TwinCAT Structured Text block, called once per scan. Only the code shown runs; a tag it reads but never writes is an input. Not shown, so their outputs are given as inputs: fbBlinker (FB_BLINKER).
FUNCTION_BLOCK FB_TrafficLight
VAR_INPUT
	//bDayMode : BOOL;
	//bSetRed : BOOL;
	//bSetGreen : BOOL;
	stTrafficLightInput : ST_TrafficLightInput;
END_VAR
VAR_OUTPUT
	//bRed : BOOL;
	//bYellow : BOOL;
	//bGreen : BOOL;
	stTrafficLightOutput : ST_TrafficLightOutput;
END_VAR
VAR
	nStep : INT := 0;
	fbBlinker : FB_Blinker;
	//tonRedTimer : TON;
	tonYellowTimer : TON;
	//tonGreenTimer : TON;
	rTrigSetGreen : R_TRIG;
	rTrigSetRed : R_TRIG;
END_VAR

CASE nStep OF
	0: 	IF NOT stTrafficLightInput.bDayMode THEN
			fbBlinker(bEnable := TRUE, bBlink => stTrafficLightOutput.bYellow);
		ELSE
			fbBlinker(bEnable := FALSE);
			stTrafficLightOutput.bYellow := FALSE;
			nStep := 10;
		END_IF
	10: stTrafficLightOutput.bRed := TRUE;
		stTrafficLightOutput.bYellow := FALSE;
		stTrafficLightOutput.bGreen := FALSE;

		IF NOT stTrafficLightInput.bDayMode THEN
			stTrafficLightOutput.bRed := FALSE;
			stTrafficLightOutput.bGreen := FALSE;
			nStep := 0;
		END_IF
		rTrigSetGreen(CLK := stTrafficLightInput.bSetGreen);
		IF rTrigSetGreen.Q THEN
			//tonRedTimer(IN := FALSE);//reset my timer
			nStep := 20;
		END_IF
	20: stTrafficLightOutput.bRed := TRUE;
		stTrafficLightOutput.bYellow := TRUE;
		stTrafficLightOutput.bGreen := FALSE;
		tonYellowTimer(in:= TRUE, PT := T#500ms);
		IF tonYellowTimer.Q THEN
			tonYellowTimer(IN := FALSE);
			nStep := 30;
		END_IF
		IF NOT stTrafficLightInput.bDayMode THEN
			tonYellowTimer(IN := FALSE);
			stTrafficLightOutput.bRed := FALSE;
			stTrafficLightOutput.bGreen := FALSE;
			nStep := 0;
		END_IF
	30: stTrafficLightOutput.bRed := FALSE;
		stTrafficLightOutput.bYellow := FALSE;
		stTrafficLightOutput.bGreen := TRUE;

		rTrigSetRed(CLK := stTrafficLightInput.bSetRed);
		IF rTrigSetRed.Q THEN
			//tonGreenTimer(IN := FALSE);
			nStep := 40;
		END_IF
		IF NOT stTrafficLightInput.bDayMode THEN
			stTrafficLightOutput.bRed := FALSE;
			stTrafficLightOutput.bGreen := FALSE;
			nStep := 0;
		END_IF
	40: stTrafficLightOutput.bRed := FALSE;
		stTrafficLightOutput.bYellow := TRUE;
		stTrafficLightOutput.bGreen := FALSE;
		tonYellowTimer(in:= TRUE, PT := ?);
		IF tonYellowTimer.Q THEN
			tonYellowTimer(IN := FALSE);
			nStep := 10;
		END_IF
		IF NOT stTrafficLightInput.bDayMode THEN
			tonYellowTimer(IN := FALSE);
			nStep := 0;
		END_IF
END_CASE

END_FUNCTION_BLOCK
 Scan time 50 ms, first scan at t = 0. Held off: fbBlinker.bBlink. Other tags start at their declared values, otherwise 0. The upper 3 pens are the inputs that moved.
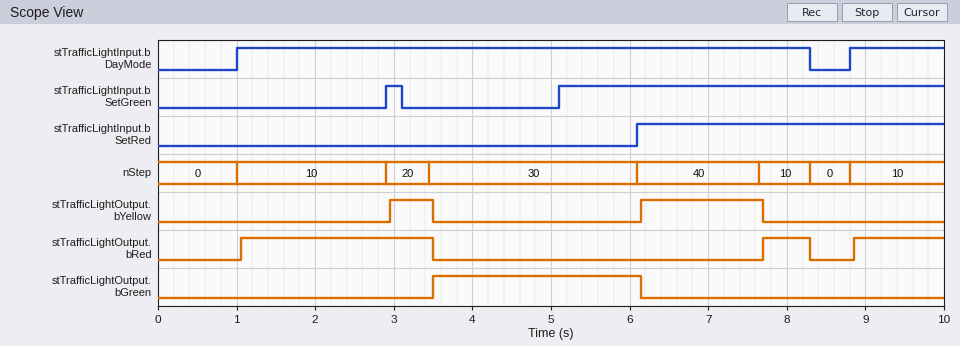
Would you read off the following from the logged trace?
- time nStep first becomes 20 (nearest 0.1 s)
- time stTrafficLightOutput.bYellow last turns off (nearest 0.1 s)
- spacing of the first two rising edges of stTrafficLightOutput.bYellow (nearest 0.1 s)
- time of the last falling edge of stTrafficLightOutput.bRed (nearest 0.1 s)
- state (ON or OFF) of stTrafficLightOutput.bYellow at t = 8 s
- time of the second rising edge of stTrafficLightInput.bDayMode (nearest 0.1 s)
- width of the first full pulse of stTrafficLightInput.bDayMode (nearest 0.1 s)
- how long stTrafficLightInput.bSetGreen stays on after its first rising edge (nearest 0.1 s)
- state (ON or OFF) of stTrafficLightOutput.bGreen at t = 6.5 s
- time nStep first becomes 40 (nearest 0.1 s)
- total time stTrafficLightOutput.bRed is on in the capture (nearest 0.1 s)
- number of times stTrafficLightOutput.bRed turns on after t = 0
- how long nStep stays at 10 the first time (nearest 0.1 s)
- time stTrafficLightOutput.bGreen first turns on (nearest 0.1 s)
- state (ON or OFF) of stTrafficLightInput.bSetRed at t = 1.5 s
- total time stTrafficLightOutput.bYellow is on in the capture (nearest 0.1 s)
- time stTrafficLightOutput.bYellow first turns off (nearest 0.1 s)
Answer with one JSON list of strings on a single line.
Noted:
["2.9 s", "7.7 s", "3.2 s", "8.3 s", "OFF", "8.8 s", "7.3 s", "0.2 s", "OFF", "6.1 s", "4.2 s", "3", "1.9 s", "3.5 s", "OFF", "2.1 s", "3.5 s"]
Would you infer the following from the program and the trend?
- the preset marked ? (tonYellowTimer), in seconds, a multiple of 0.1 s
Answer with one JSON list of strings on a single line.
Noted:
["1.5 s"]
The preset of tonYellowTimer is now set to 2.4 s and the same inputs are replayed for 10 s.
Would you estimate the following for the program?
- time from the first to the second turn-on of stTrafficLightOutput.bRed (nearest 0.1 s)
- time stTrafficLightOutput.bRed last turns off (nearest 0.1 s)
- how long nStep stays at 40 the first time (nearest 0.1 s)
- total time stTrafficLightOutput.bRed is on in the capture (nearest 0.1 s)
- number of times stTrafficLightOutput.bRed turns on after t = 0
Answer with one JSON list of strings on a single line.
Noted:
["7.8 s", "3.5 s", "2.2 s", "3.6 s", "2"]
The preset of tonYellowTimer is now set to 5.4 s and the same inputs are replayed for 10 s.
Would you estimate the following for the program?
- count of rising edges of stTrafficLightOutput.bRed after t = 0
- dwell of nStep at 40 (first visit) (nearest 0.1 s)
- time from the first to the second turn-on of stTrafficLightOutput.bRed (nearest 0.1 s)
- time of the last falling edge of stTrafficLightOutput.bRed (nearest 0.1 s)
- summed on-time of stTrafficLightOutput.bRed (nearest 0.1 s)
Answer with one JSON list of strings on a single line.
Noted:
["2", "2.2 s", "7.8 s", "3.5 s", "3.6 s"]
